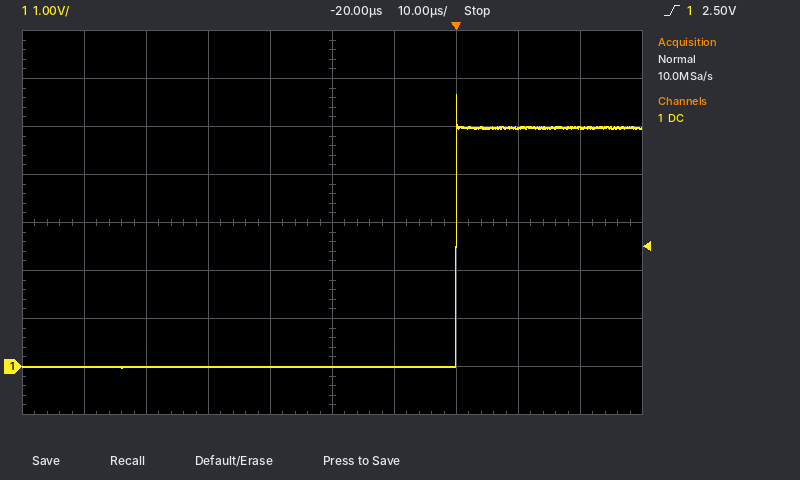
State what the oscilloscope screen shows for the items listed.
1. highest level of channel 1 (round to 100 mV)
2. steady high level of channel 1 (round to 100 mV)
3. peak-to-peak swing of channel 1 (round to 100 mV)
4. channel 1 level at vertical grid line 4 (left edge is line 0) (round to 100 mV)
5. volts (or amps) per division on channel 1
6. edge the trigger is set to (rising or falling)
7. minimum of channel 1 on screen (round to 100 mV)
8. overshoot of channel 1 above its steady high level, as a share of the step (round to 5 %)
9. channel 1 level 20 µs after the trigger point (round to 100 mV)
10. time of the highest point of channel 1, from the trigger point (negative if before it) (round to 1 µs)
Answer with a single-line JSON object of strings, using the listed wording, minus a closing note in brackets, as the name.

{"highest level of channel 1": "5.7 V", "steady high level of channel 1": "5.0 V", "peak-to-peak swing of channel 1": "5.7 V", "channel 1 level at vertical grid line 4 (left edge is line 0)": "0.0 V", "volts (or amps) per division on channel 1": "1 V", "edge the trigger is set to": "rising", "minimum of channel 1 on screen": "0.0 V", "overshoot of channel 1 above its steady high level, as a share of the step": "15 %", "channel 1 level 20 µs after the trigger point": "5.0 V", "time of the highest point of channel 1, from the trigger point (negative if before it)": "0 µs"}
